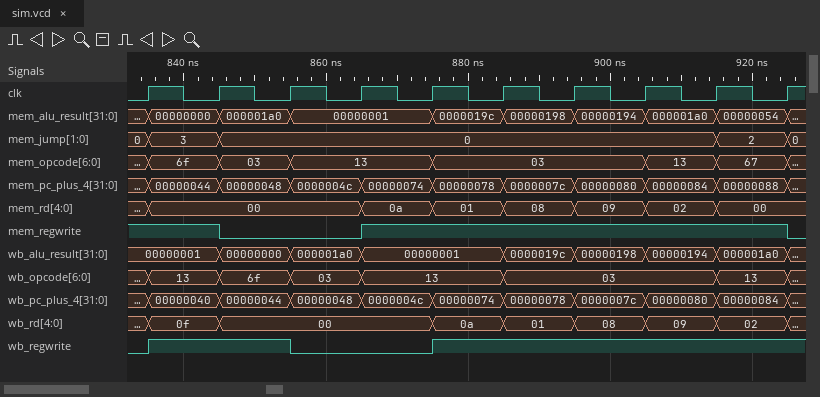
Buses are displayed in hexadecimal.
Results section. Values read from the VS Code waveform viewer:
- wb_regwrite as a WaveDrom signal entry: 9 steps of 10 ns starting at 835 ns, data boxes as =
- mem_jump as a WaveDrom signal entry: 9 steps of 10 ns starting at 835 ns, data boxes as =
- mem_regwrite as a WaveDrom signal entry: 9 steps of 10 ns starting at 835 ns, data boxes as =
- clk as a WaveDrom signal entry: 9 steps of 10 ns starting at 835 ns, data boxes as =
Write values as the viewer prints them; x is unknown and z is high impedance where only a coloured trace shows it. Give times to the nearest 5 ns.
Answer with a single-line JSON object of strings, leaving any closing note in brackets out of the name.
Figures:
{"wb_regwrite as a WaveDrom signal entry: 9 steps of 10 ns starting at 835 ns, data boxes as =": "{name: 'wb_regwrite', wave: '1.0.1....'}", "mem_jump as a WaveDrom signal entry: 9 steps of 10 ns starting at 835 ns, data boxes as =": "{name: 'mem_jump', wave: '==......=', data: '3 0 2'}", "mem_regwrite as a WaveDrom signal entry: 9 steps of 10 ns starting at 835 ns, data boxes as =": "{name: 'mem_regwrite', wave: '10.1.....'}", "clk as a WaveDrom signal entry: 9 steps of 10 ns starting at 835 ns, data boxes as =": "{name: 'clk', wave: 'p........'}"}
